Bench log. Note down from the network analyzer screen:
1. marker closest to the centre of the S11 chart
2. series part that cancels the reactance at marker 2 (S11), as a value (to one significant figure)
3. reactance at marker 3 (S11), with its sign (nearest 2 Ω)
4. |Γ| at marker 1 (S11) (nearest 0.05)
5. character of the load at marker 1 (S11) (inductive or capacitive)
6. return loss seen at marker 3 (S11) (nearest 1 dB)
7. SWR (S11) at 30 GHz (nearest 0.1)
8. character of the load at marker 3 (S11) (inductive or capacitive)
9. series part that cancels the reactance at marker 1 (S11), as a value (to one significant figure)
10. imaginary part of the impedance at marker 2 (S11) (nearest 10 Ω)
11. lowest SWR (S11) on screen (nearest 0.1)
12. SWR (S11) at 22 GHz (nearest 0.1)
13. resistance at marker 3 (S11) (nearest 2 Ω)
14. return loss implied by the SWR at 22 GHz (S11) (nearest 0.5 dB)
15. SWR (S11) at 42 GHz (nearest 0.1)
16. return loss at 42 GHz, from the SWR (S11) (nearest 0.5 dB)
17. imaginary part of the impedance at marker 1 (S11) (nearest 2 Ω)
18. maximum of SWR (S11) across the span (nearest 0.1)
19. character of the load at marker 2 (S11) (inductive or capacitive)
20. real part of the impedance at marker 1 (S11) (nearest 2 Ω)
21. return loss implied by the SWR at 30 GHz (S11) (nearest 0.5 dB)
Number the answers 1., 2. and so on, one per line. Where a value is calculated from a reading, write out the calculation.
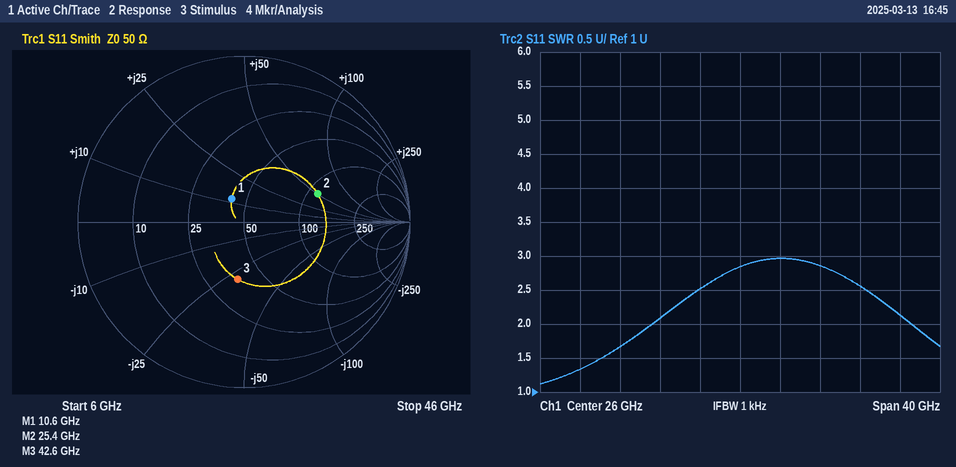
1. marker 1
2. C = 1/(2π × 25.4 GHz × 50 Ω) ≈ 125 fF, so 100 fF to one significant figure
3. -28 Ω
4. 0.15
5. inductive
6. 9 dB
7. 3.0
8. capacitive
9. C = 1/(2π × 10.6 GHz × 12 Ω) ≈ 1 pF
10. +50 Ω
11. 1.1
12. 2.5
13. 36 Ω
14. −20 log10((2.5 − 1)/(2.5 + 1)) ≈ 7.36 dB, so 7.5 dB to the nearest 0.5 dB
15. 2.1
16. −20 log10((2.1 − 1)/(2.1 + 1)) ≈ 9.0 dB
17. +12 Ω
18. 3.0
19. inductive
20. 42 Ω
21. −20 log10((3 − 1)/(3 + 1)) ≈ 6.0 dB
